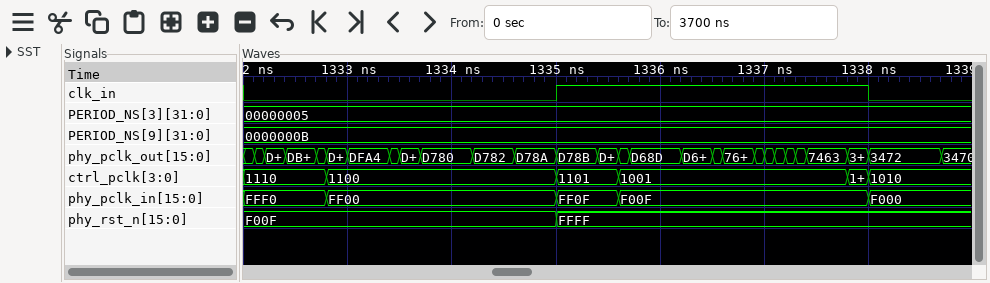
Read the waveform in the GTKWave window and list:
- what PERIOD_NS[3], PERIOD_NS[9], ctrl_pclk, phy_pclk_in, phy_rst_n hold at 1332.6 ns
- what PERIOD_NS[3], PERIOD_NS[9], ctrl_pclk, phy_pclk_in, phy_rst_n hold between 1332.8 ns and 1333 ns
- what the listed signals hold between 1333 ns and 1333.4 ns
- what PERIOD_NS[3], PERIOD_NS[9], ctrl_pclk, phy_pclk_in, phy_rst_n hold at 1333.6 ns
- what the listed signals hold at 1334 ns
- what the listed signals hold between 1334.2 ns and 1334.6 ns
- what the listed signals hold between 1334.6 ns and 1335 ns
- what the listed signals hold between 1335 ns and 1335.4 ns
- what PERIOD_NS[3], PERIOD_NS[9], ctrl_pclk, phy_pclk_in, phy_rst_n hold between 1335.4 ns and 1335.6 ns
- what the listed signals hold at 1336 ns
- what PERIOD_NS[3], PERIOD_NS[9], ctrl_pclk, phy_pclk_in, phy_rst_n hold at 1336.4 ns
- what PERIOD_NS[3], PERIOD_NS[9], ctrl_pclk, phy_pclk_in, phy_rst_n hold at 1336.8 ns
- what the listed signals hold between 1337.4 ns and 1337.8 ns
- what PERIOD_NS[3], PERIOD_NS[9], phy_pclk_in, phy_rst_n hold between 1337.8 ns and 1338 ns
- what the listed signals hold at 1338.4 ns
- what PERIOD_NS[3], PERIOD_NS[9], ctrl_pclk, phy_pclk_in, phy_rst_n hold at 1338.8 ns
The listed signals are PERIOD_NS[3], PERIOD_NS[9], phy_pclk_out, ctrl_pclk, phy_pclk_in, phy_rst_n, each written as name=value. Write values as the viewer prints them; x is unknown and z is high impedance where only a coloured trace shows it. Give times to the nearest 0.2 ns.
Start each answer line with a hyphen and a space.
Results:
- PERIOD_NS[3]=00000005, PERIOD_NS[9]=0000000B, ctrl_pclk=1110, phy_pclk_in=FFF0, phy_rst_n=F00F
- PERIOD_NS[3]=00000005, PERIOD_NS[9]=0000000B, ctrl_pclk=1100, phy_pclk_in=FF00, phy_rst_n=F00F
- PERIOD_NS[3]=00000005, PERIOD_NS[9]=0000000B, phy_pclk_out=DFA4, ctrl_pclk=1100, phy_pclk_in=FF00, phy_rst_n=F00F
- PERIOD_NS[3]=00000005, PERIOD_NS[9]=0000000B, ctrl_pclk=1100, phy_pclk_in=FF00, phy_rst_n=F00F
- PERIOD_NS[3]=00000005, PERIOD_NS[9]=0000000B, phy_pclk_out=D780, ctrl_pclk=1100, phy_pclk_in=FF00, phy_rst_n=F00F
- PERIOD_NS[3]=00000005, PERIOD_NS[9]=0000000B, phy_pclk_out=D782, ctrl_pclk=1100, phy_pclk_in=FF00, phy_rst_n=F00F
- PERIOD_NS[3]=00000005, PERIOD_NS[9]=0000000B, phy_pclk_out=D78A, ctrl_pclk=1100, phy_pclk_in=FF00, phy_rst_n=F00F
- PERIOD_NS[3]=00000005, PERIOD_NS[9]=0000000B, phy_pclk_out=D78B, ctrl_pclk=1101, phy_pclk_in=FF0F, phy_rst_n=FFFF
- PERIOD_NS[3]=00000005, PERIOD_NS[9]=0000000B, ctrl_pclk=1101, phy_pclk_in=FF0F, phy_rst_n=FFFF
- PERIOD_NS[3]=00000005, PERIOD_NS[9]=0000000B, phy_pclk_out=D68D, ctrl_pclk=1001, phy_pclk_in=F00F, phy_rst_n=FFFF
- PERIOD_NS[3]=00000005, PERIOD_NS[9]=0000000B, ctrl_pclk=1001, phy_pclk_in=F00F, phy_rst_n=FFFF
- PERIOD_NS[3]=00000005, PERIOD_NS[9]=0000000B, ctrl_pclk=1001, phy_pclk_in=F00F, phy_rst_n=FFFF
- PERIOD_NS[3]=00000005, PERIOD_NS[9]=0000000B, phy_pclk_out=7463, ctrl_pclk=1001, phy_pclk_in=F00F, phy_rst_n=FFFF
- PERIOD_NS[3]=00000005, PERIOD_NS[9]=0000000B, phy_pclk_in=F00F, phy_rst_n=FFFF
- PERIOD_NS[3]=00000005, PERIOD_NS[9]=0000000B, phy_pclk_out=3472, ctrl_pclk=1010, phy_pclk_in=F000, phy_rst_n=FFFF
- PERIOD_NS[3]=00000005, PERIOD_NS[9]=0000000B, ctrl_pclk=1010, phy_pclk_in=F000, phy_rst_n=FFFF
